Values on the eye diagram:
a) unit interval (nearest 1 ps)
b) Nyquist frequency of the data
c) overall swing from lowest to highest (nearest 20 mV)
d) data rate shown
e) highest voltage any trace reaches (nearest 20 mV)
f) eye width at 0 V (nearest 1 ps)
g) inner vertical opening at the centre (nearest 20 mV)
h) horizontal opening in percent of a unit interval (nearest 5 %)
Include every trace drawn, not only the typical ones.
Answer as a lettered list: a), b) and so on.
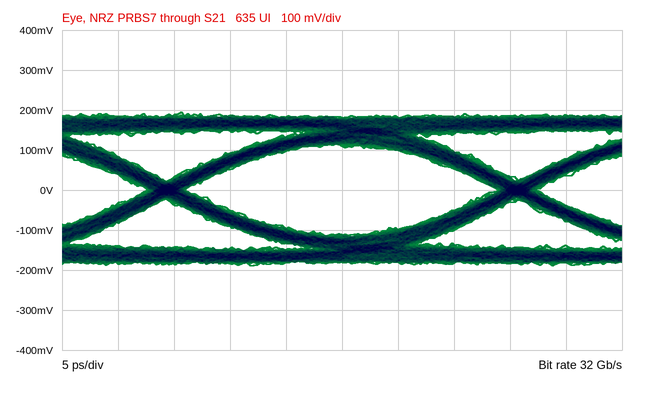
a) 31 ps
b) 16 GHz
c) 380 mV
d) 32 Gb/s
e) 200 mV
f) 28 ps
g) 220 mV
h) 90 %
